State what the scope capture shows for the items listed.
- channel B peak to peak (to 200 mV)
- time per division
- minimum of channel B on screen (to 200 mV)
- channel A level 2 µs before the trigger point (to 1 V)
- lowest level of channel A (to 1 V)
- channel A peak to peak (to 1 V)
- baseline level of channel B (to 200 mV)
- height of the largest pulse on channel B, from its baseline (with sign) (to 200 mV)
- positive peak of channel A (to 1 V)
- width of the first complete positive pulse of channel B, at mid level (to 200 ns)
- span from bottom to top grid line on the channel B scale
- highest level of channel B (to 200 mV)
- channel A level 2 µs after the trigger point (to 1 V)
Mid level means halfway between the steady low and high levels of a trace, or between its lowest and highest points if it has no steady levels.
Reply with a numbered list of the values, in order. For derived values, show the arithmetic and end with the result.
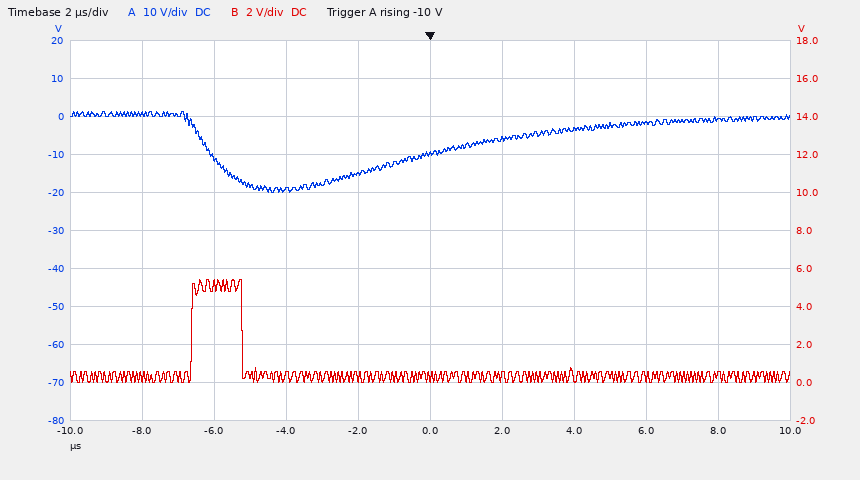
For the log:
1. 5.4 V − (0.0 V) = 5.4 V
2. 2 µs
3. 0.0 V
4. -15 V
5. -20 V
6. 1 V − (-20 V) = 21 V
7. 400 mV
8. 5.4 V − (400 mV) = +5.0 V
9. 1 V
10. 1.4 µs
11. 20 V
12. 5.4 V
13. -6 V
